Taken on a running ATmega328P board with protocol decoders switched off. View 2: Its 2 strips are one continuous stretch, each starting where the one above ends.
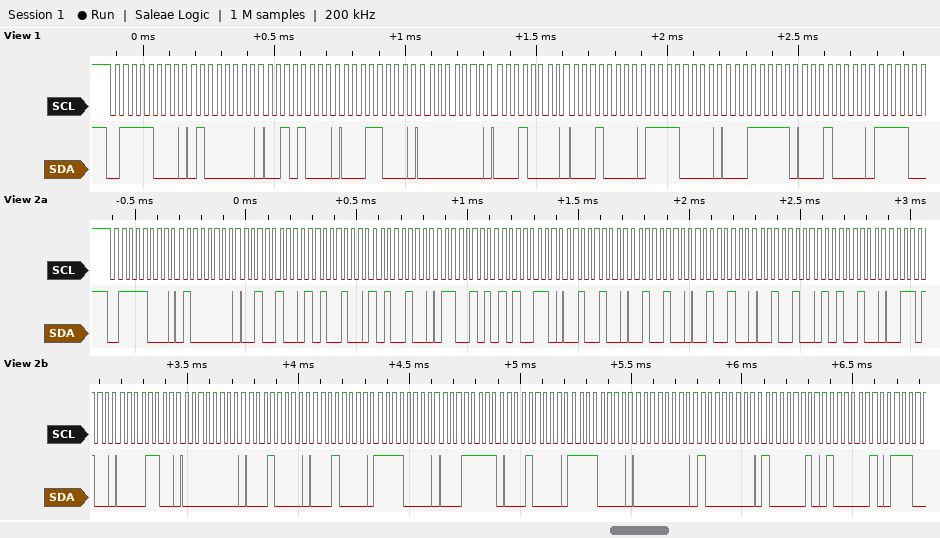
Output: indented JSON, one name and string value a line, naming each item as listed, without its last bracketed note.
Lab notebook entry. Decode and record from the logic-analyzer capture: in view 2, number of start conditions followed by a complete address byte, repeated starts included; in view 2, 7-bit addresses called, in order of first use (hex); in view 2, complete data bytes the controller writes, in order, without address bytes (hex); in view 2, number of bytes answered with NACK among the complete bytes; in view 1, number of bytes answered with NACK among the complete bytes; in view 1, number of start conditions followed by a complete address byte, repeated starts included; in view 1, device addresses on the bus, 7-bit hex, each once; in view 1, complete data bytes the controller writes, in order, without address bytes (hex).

{
  "in view 2, number of start conditions followed by a complete address byte, repeated starts included": "1",
  "in view 2, 7-bit addresses called, in order of first use": "0x3C",
  "in view 2, complete data bytes the controller writes, in order, without address bytes": "40 24 A4 A4 65 A6 24 24 24 24 A4 34 0C 00 10 10 F0 1F 10 F0 00 80 82 82",
  "in view 2, number of bytes answered with NACK among the complete bytes": "0",
  "in view 1, number of bytes answered with NACK among the complete bytes": "0",
  "in view 1, number of start conditions followed by a complete address byte, repeated starts included": "1",
  "in view 1, device addresses on the bus, 7-bit hex, each once": "0x3C",
  "in view 1, complete data bytes the controller writes, in order, without address bytes": "40 28 18 00 10 10 F0 1F 10"
}
